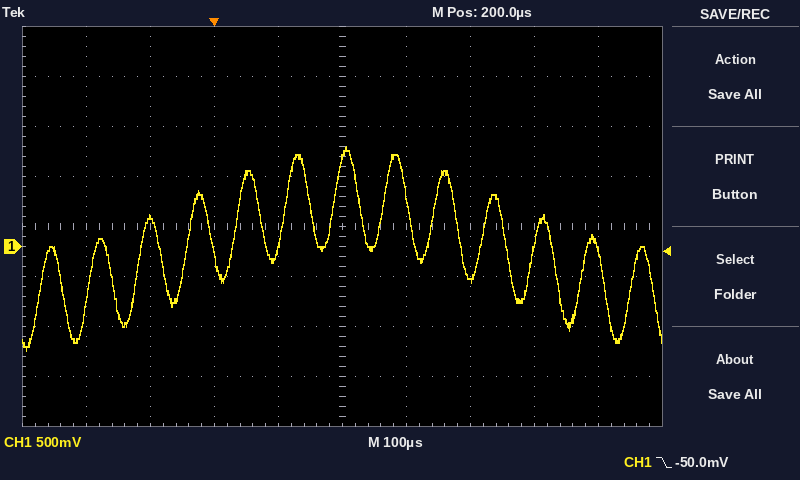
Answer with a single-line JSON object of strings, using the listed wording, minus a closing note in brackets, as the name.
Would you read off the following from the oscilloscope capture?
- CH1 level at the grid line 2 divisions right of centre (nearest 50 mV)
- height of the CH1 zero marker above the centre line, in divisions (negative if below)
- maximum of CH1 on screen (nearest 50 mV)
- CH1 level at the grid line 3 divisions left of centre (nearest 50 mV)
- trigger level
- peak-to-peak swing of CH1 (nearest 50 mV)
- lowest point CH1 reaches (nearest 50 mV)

{"CH1 level at the grid line 2 divisions right of centre": "-300 mV", "height of the CH1 zero marker above the centre line, in divisions": "-0.4 div", "maximum of CH1 on screen": "1.00 V", "CH1 level at the grid line 3 divisions left of centre": "300 mV", "trigger level": "-50.0 mV", "peak-to-peak swing of CH1": "2.05 V", "lowest point CH1 reaches": "-1.05 V"}
